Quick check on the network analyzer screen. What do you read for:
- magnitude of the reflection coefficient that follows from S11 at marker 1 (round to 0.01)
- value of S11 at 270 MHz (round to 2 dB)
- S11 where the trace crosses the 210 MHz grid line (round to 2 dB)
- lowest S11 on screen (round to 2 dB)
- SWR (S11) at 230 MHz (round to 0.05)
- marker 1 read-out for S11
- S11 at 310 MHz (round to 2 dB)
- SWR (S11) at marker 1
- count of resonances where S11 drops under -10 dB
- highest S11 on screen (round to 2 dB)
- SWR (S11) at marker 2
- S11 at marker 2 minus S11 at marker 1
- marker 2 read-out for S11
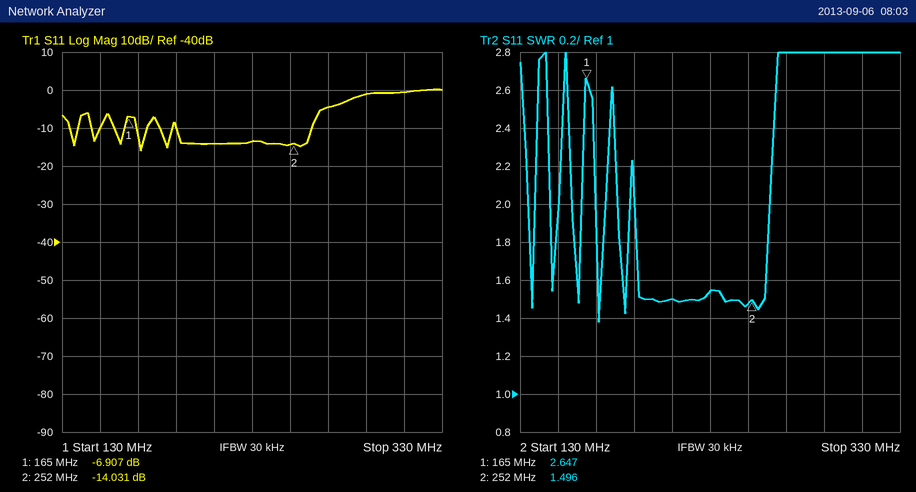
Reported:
0.45
-4 dB
-14 dB
-16 dB
1.55
-6.907 dB
0 dB
2.647
6
0 dB
1.496
-7.124 dB
-14.031 dB
